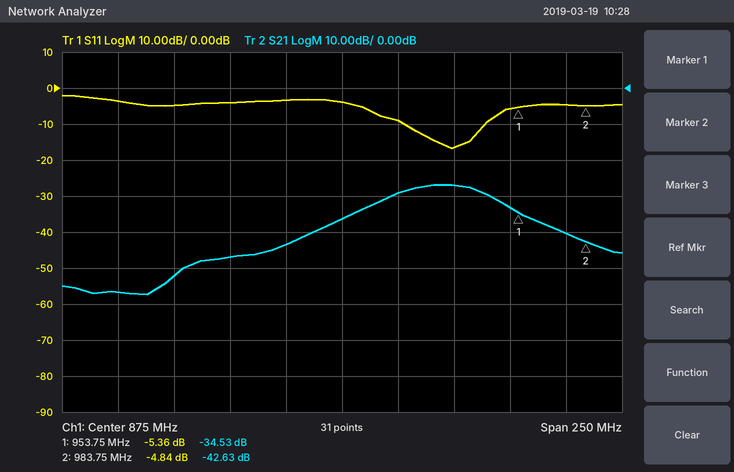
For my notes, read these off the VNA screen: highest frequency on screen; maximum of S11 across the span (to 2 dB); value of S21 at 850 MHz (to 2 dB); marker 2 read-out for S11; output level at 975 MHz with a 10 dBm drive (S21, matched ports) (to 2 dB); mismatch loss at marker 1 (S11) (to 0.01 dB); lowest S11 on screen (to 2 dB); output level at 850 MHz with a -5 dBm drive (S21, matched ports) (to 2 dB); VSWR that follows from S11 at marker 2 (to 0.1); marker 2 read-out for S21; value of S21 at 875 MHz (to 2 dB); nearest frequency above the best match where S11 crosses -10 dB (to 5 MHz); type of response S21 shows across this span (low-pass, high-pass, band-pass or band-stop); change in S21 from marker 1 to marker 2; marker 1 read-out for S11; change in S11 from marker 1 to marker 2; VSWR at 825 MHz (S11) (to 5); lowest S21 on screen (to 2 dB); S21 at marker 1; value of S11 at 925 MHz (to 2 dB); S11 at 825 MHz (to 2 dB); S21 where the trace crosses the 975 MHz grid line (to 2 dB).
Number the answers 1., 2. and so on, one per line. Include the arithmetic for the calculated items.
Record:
1. 1 GHz
2. -2 dB
3. -44 dB
4. -4.84 dB
5. 10 dBm + (-40 dB) = -30 dBm
6. −10 log10(1 − 10^(-5.36/10)) ≈ 1.49 dB
7. -16 dB
8. -5 dBm + (-44 dB) = -48 dBm
9. (1 + 0.5728)/(1 − 0.5728) ≈ 3.7
10. -42.63 dB
11. -36 dB
12. 940 MHz
13. band-pass
14. -42.63 − (-34.53) = -8.10 dB
15. -5.36 dB
16. -4.84 − (-5.36) = 0.52 dB
17. |Γ| = 10^(-4/20) = 0.6310; VSWR = (1 + 0.6310)/(1 − 0.6310) ≈ 4.42, so 5 to the nearest 5
18. -58 dB
19. -34.53 dB
20. -16 dB
21. -4 dB
22. -40 dB
